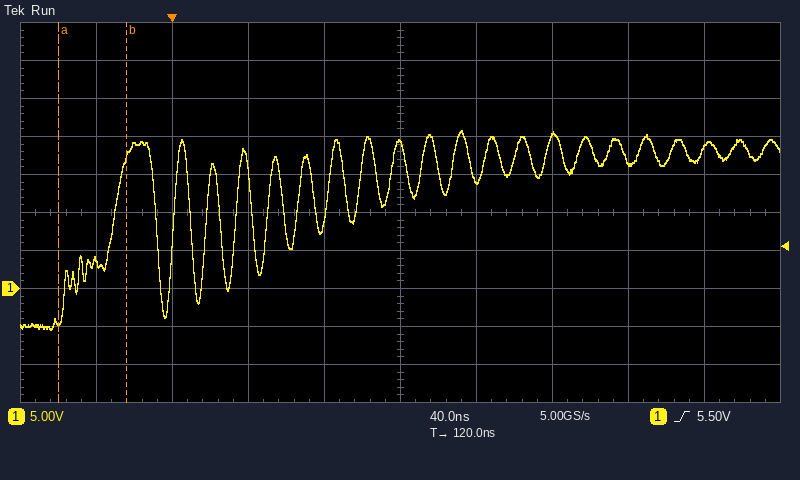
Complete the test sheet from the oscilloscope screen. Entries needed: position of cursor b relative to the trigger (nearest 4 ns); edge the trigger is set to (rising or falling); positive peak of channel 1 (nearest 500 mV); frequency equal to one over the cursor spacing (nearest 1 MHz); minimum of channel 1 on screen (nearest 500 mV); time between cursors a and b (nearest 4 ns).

-24 ns
rising
21.0 V
28 MHz
-5.5 V
36 ns
